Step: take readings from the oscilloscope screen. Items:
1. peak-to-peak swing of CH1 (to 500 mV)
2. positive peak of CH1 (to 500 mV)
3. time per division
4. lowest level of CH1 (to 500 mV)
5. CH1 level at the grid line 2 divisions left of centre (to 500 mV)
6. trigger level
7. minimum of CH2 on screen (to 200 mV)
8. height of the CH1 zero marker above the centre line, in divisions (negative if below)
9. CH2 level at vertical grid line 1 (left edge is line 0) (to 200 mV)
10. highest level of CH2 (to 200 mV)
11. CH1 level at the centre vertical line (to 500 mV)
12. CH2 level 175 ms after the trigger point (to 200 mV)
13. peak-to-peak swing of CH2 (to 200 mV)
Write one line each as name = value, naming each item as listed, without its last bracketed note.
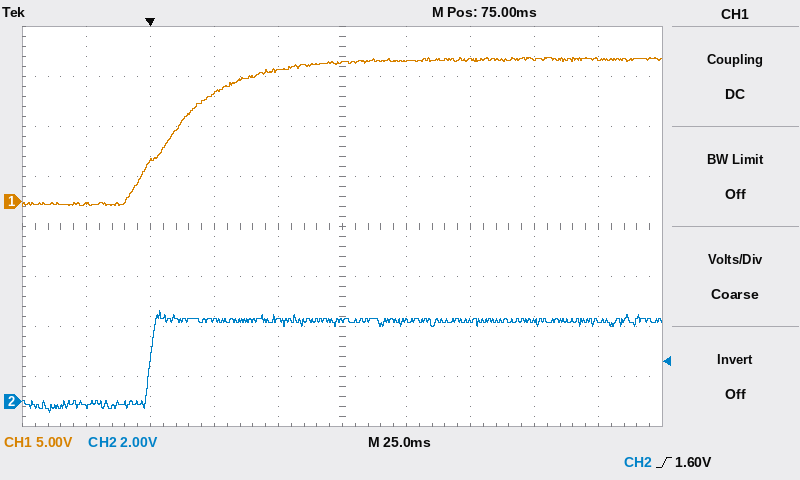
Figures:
peak-to-peak swing of CH1 = 15.0 V
positive peak of CH1 = 14.5 V
time per division = 25 ms
lowest level of CH1 = -500 mV
CH1 level at the grid line 2 divisions left of centre = 11.0 V
trigger level = 1.60 V
minimum of CH2 on screen = -400 mV
height of the CH1 zero marker above the centre line, in divisions = +0.5 div
CH2 level at vertical grid line 1 (left edge is line 0) = -200 mV
highest level of CH2 = 3.6 V
CH1 level at the centre vertical line = 14.0 V
CH2 level 175 ms after the trigger point = 3.2 V
peak-to-peak swing of CH2 = 4.0 V
